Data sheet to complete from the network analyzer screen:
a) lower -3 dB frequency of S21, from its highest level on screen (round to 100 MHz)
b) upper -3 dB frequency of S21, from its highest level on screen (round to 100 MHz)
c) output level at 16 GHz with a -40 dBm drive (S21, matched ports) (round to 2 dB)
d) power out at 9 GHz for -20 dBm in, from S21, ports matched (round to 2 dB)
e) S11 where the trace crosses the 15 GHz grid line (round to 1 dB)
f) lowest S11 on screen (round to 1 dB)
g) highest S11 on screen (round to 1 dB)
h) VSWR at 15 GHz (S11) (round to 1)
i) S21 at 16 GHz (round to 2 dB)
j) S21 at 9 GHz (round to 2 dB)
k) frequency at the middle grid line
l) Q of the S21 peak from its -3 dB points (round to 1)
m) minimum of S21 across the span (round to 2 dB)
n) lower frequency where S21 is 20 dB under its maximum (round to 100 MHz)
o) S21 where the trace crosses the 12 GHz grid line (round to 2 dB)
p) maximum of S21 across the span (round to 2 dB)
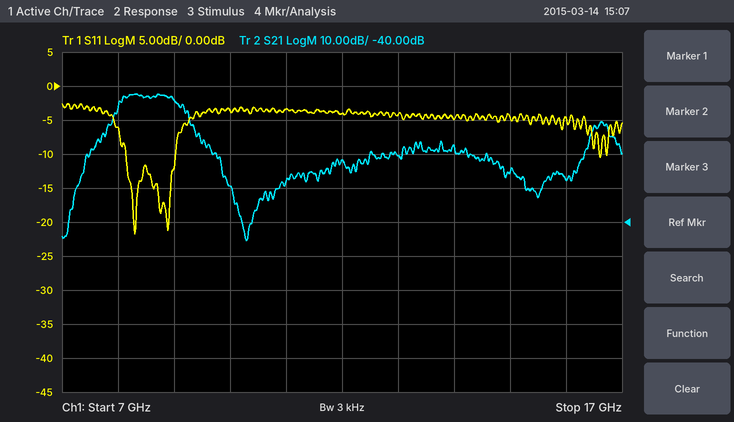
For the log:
8.0 GHz
9.1 GHz
-68 dBm
-24 dBm
-5 dB
-22 dB
-3 dB
4
-28 dB
-4 dB
12 GHz
8
-46 dB
7.4 GHz
-22 dB
-2 dB
